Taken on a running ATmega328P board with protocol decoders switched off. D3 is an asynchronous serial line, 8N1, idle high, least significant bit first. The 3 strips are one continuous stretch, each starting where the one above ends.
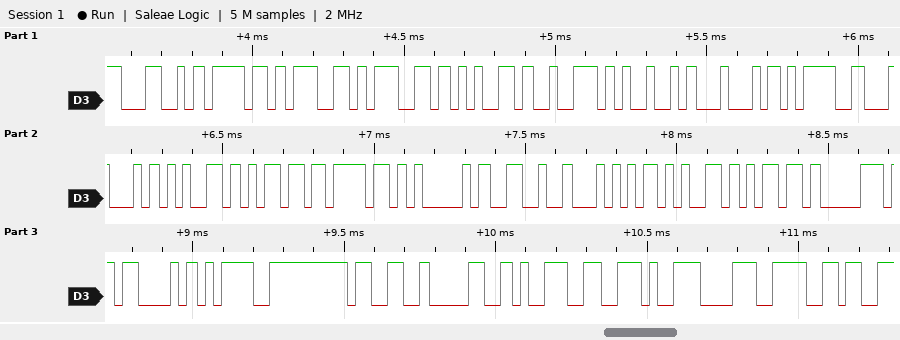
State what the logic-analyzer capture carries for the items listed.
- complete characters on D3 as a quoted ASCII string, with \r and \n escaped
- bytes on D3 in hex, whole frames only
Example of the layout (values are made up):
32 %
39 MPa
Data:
"LoggerID=DemoA&TempC=309.86"
0x4C 0x6F 0x67 0x67 0x65 0x72 0x49 0x44 0x3D 0x44 0x65 0x6D 0x6F 0x41 0x26 0x54 0x65 0x6D 0x70 0x43 0x3D 0x33 0x30 0x39 0x2E 0x38 0x36
